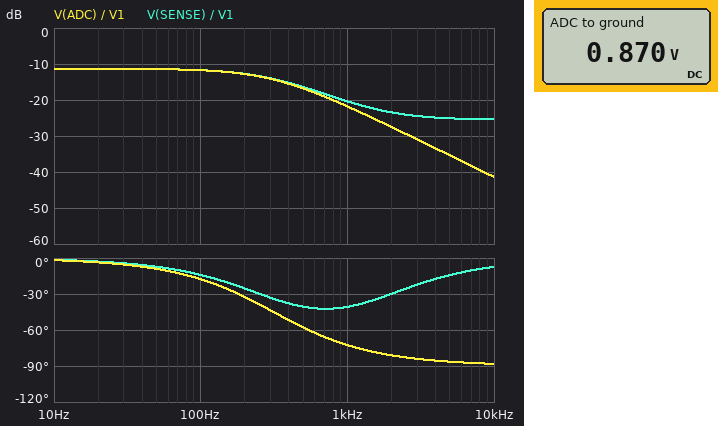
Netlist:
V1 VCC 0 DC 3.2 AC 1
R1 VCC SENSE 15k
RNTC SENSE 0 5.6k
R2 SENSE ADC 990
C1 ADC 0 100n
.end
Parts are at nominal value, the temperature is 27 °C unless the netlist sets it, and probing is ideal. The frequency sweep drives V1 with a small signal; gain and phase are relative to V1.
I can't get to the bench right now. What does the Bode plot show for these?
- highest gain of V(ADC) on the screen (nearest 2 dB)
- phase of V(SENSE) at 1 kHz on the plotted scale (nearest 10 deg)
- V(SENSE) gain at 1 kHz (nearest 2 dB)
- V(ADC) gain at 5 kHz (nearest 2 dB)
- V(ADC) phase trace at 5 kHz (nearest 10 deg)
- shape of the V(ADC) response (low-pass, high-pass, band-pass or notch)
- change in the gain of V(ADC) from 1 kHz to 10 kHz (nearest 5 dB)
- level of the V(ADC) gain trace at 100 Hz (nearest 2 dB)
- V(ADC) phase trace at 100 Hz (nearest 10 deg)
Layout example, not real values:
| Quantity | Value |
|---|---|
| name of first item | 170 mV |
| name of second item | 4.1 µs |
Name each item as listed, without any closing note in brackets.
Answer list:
| Quantity | Value |
|---|---|
| highest gain of V(ADC) on the screen | -12 dB |
| phase of V(SENSE) at 1 kHz on the plotted scale | -40 deg |
| V(SENSE) gain at 1 kHz | -20 dB |
| V(ADC) gain at 5 kHz | -36 dB |
| V(ADC) phase trace at 5 kHz | -90 deg |
| shape of the V(ADC) response | low-pass |
| change in the gain of V(ADC) from 1 kHz to 10 kHz | -20 dB |
| level of the V(ADC) gain trace at 100 Hz | -12 dB |
| V(ADC) phase trace at 100 Hz | -20 deg |
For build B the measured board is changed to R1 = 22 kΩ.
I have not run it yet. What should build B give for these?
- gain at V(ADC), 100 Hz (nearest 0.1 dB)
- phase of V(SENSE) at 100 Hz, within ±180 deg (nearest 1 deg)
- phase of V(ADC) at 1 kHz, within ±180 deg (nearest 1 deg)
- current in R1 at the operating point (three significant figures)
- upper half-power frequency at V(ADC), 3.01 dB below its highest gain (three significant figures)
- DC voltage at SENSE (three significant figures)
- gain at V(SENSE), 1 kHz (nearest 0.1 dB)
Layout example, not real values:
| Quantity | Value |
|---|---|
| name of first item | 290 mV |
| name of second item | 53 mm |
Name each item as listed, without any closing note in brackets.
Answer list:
| Quantity | Value |
|---|---|
| gain at V(ADC), 100 Hz | -14.3 dB |
| phase of V(SENSE) at 100 Hz, within ±180 deg | -15 deg |
| phase of V(ADC) at 1 kHz, within ±180 deg | -74 deg |
| current in R1 at the operating point | 116 µA |
| upper half-power frequency at V(ADC), 3.01 dB below its highest gain | 292 Hz |
| DC voltage at SENSE | 649 mV |
| gain at V(SENSE), 1 kHz | -23.5 dB |
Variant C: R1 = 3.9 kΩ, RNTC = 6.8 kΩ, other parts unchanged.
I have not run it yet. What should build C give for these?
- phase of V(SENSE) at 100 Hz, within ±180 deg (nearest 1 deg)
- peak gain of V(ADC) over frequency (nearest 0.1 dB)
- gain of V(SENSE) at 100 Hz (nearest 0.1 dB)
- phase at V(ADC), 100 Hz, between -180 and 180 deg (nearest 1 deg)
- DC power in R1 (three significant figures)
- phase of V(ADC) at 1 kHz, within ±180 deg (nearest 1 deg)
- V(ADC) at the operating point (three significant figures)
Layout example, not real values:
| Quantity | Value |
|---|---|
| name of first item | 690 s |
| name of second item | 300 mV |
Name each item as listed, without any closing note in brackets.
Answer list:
| Quantity | Value |
|---|---|
| phase of V(SENSE) at 100 Hz, within ±180 deg | -9 deg |
| peak gain of V(ADC) over frequency | -3.9 dB |
| gain of V(SENSE) at 100 Hz | -4.1 dB |
| phase at V(ADC), 100 Hz, between -180 and 180 deg | -12 deg |
| DC power in R1 | 349 µW |
| phase of V(ADC) at 1 kHz, within ±180 deg | -65 deg |
| V(ADC) at the operating point | 2.03 V |
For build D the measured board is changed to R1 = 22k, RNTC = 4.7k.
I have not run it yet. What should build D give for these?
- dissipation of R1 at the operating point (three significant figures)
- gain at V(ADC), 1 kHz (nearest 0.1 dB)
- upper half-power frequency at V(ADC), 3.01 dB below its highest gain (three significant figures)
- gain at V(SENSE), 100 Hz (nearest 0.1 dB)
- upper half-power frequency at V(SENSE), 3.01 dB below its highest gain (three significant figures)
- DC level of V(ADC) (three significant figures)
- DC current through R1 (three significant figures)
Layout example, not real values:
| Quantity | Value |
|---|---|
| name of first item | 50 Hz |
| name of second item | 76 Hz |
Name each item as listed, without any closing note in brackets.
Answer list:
| Quantity | Value |
|---|---|
| dissipation of R1 at the operating point | 316 µW |
| gain at V(ADC), 1 kHz | -25.2 dB |
| upper half-power frequency at V(ADC), 3.01 dB below its highest gain | 327 Hz |
| gain at V(SENSE), 100 Hz | -15.5 dB |
| upper half-power frequency at V(SENSE), 3.01 dB below its highest gain | 342 Hz |
| DC level of V(ADC) | 563 mV |
| DC current through R1 | 120 µA |
